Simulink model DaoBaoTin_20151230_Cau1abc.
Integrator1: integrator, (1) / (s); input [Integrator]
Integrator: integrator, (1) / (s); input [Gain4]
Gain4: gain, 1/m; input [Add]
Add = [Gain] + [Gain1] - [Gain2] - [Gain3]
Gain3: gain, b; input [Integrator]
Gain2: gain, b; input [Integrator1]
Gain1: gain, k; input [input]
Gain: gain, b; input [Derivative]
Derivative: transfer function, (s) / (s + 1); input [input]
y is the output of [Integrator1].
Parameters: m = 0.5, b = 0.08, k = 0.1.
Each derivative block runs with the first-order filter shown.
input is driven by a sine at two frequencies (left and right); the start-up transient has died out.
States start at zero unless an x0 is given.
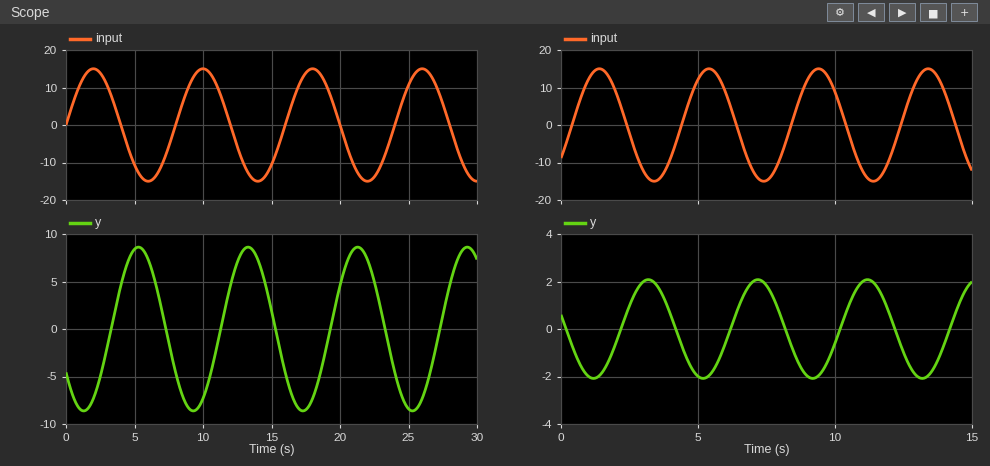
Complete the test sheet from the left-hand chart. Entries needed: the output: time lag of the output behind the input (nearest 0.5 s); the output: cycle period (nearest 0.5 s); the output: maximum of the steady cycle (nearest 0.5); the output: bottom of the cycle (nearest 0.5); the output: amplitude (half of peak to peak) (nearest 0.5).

3.5 s
8.0 s
8.5
-8.5
8.5
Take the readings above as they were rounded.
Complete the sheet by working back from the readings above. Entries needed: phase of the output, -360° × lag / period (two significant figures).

-160°
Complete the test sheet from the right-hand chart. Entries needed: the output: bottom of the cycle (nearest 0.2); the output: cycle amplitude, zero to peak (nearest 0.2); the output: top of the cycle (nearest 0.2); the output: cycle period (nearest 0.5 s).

-2.0
2.0
2.0
4.0 s
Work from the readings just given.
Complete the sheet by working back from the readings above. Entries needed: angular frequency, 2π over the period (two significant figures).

1.6 rad/s
